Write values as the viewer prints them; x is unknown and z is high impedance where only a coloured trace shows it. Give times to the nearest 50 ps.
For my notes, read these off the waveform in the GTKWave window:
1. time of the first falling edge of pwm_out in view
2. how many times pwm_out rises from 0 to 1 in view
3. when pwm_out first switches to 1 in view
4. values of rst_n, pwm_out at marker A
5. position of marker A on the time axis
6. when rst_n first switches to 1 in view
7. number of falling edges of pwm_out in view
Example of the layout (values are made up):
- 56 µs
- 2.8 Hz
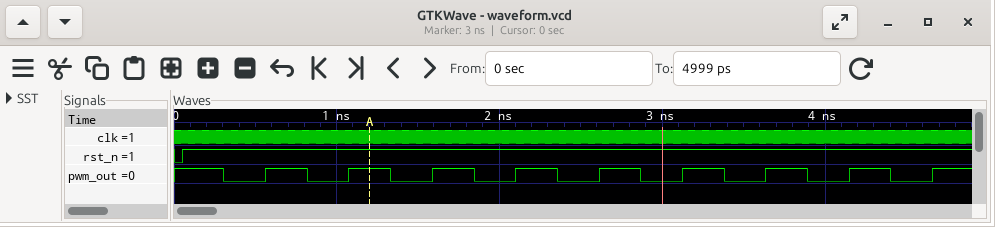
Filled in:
- 300 ps
- 9
- 550 ps
- rst_n=1, pwm_out=1
- 1200 ps
- 50 ps
- 9
